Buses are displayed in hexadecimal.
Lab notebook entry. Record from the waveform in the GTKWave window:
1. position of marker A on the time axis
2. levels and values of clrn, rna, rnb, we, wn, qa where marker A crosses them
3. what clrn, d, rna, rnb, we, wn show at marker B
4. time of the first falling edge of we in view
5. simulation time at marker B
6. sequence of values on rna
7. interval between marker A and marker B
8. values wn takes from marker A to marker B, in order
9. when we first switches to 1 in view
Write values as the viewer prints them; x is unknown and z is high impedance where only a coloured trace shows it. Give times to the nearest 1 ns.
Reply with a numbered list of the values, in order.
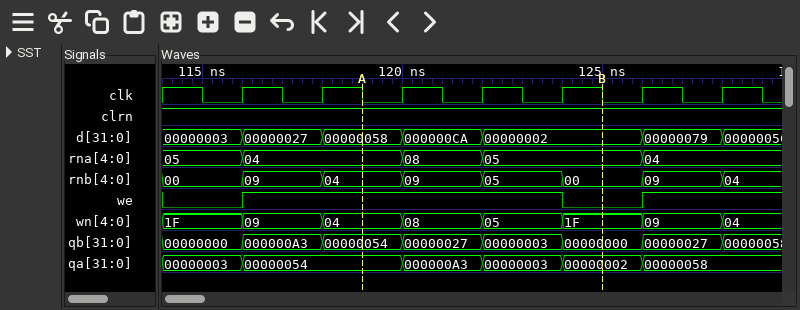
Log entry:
1. 119 ns
2. clrn=1, rna=04, rnb=04, we=1, wn=04, qa=00000054
3. clrn=1, d=00000002, rna=05, rnb=00, we=0, wn=1F
4. 124 ns
5. 125 ns
6. 05, 04, 08, 05, 04
7. 6 ns
8. 04, 08, 05, 1F
9. 116 ns
